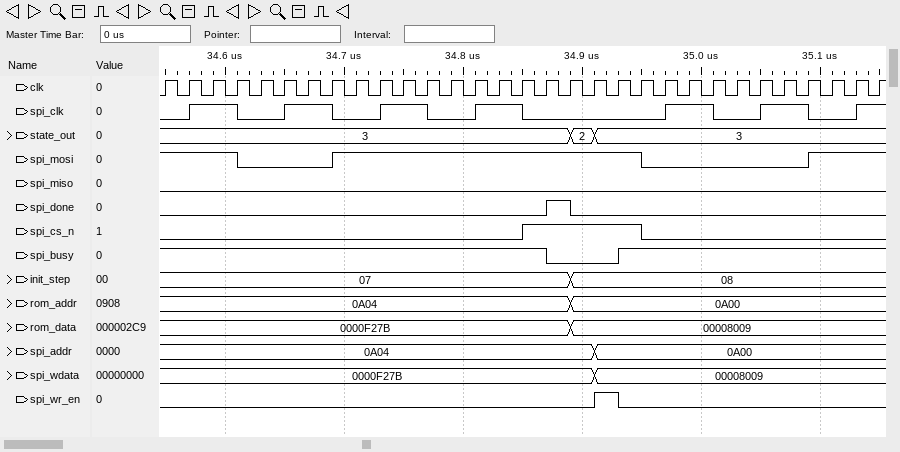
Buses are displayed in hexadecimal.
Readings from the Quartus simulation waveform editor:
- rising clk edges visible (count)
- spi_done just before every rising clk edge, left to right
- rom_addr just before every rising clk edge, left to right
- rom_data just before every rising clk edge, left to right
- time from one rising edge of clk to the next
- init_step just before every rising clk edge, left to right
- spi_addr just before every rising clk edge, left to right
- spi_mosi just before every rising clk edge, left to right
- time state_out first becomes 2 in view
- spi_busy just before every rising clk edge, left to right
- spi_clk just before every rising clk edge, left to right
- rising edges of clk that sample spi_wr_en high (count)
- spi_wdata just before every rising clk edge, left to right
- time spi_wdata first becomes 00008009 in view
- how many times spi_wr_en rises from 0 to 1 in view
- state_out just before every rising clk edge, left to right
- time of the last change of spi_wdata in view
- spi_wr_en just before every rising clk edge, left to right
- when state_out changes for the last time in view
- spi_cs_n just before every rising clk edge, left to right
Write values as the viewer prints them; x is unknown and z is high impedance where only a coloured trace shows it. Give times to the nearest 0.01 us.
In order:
31
0 0 0 0 0 0 0 0 0 0 0 0 0 0 0 0 0 1 0 0 0 0 0 0 0 0 0 0 0 0 0
0A04, 0A04, 0A04, 0A04, 0A04, 0A04, 0A04, 0A04, 0A04, 0A04, 0A04, 0A04, 0A04, 0A04, 0A04, 0A04, 0A04, 0A04, 0A00, 0A00, 0A00, 0A00, 0A00, 0A00, 0A00, 0A00, 0A00, 0A00, 0A00, 0A00, 0A00
0000F27B, 0000F27B, 0000F27B, 0000F27B, 0000F27B, 0000F27B, 0000F27B, 0000F27B, 0000F27B, 0000F27B, 0000F27B, 0000F27B, 0000F27B, 0000F27B, 0000F27B, 0000F27B, 0000F27B, 0000F27B, 00008009, 00008009, 00008009, 00008009, 00008009, 00008009, 00008009, 00008009, 00008009, 00008009, 00008009, 00008009, 00008009
0.02 us
07, 07, 07, 07, 07, 07, 07, 07, 07, 07, 07, 07, 07, 07, 07, 07, 07, 07, 08, 08, 08, 08, 08, 08, 08, 08, 08, 08, 08, 08, 08
0A04, 0A04, 0A04, 0A04, 0A04, 0A04, 0A04, 0A04, 0A04, 0A04, 0A04, 0A04, 0A04, 0A04, 0A04, 0A04, 0A04, 0A04, 0A04, 0A00, 0A00, 0A00, 0A00, 0A00, 0A00, 0A00, 0A00, 0A00, 0A00, 0A00, 0A00
1 1 1 1 0 0 0 0 1 1 1 1 1 1 1 1 1 1 1 1 1 0 0 0 0 0 0 0 1 1 1
34.89 us
1 1 1 1 1 1 1 1 1 1 1 1 1 1 1 1 1 0 0 0 1 1 1 1 1 1 1 1 1 1 1
0 0 1 1 0 0 1 1 0 0 1 1 0 0 1 1 0 0 0 0 0 0 1 1 0 0 1 1 0 0 1
1
0000F27B, 0000F27B, 0000F27B, 0000F27B, 0000F27B, 0000F27B, 0000F27B, 0000F27B, 0000F27B, 0000F27B, 0000F27B, 0000F27B, 0000F27B, 0000F27B, 0000F27B, 0000F27B, 0000F27B, 0000F27B, 0000F27B, 00008009, 00008009, 00008009, 00008009, 00008009, 00008009, 00008009, 00008009, 00008009, 00008009, 00008009, 00008009
34.91 us
1
3, 3, 3, 3, 3, 3, 3, 3, 3, 3, 3, 3, 3, 3, 3, 3, 3, 3, 2, 3, 3, 3, 3, 3, 3, 3, 3, 3, 3, 3, 3
34.91 us
0 0 0 0 0 0 0 0 0 0 0 0 0 0 0 0 0 0 0 1 0 0 0 0 0 0 0 0 0 0 0
34.91 us
0 0 0 0 0 0 0 0 0 0 0 0 0 0 0 0 1 1 1 1 1 0 0 0 0 0 0 0 0 0 0
